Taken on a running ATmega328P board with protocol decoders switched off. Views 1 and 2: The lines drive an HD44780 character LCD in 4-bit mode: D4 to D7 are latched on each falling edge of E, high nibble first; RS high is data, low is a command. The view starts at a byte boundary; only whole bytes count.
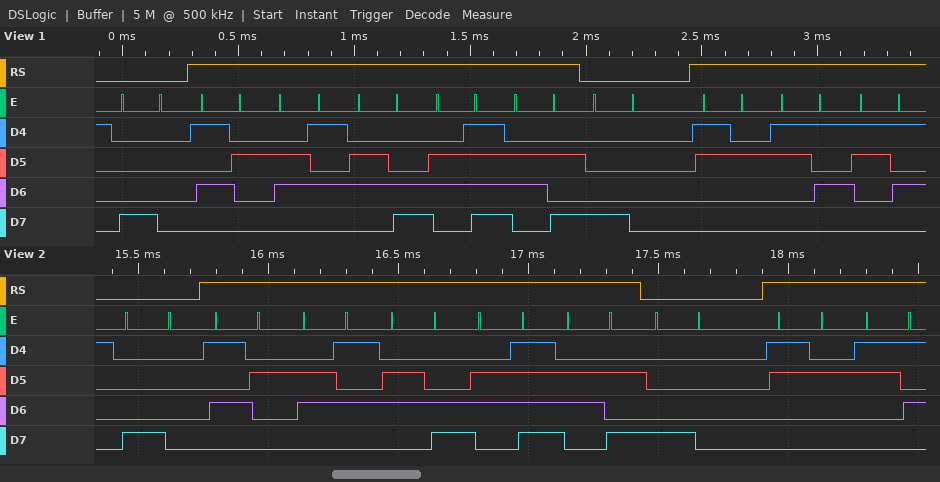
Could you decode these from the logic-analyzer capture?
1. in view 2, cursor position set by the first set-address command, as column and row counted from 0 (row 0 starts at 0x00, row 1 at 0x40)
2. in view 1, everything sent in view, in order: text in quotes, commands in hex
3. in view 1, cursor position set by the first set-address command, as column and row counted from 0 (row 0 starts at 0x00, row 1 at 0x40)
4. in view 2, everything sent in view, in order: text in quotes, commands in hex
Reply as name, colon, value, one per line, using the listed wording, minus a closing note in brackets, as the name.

in view 2, cursor position set by the first set-address command, as column and row counted from 0: column 0, row 0
in view 1, everything sent in view, in order: text in quotes, commands in hex: 0x80 "Reloj" 0x80 "255"
in view 1, cursor position set by the first set-address command, as column and row counted from 0: column 0, row 0
in view 2, everything sent in view, in order: text in quotes, commands in hex: 0x80 "Reloj" 0x80 "25"
